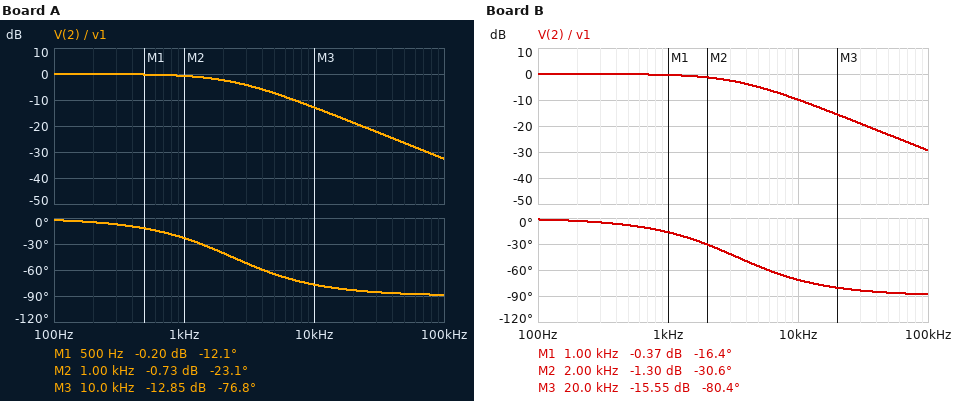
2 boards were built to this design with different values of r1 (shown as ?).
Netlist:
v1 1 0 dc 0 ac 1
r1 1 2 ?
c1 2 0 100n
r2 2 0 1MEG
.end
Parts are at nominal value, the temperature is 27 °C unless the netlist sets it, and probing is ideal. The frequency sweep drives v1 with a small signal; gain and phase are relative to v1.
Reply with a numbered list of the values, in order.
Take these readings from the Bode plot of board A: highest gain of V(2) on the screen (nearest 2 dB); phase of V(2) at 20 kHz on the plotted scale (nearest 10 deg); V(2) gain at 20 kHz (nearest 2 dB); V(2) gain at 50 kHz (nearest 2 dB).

1. 0 dB
2. -80 deg
3. -18 dB
4. -26 dB
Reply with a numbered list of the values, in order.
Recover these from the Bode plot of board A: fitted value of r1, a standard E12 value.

1. 680 Ω
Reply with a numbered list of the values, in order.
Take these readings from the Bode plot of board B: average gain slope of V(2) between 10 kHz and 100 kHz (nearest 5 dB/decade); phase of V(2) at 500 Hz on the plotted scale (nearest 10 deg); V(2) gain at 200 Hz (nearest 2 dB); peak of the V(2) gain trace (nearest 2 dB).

1. -20 dB/decade
2. -10 deg
3. 0 dB
4. 0 dB
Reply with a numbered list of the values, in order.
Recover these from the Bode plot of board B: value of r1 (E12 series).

1. 470 Ω
